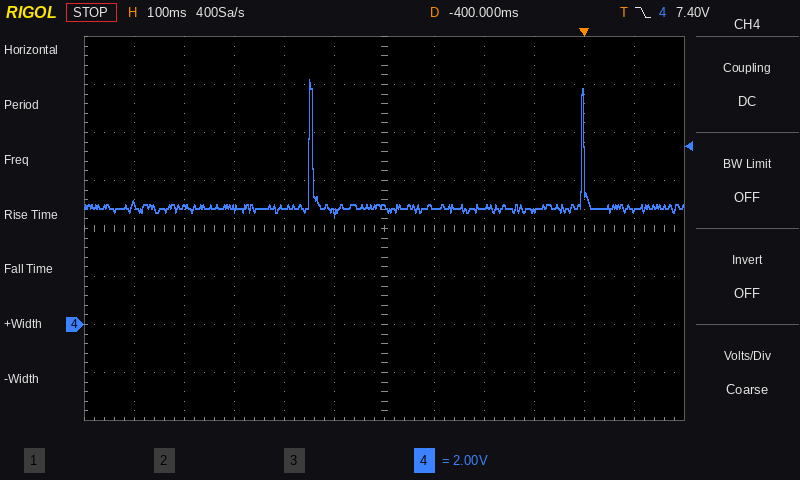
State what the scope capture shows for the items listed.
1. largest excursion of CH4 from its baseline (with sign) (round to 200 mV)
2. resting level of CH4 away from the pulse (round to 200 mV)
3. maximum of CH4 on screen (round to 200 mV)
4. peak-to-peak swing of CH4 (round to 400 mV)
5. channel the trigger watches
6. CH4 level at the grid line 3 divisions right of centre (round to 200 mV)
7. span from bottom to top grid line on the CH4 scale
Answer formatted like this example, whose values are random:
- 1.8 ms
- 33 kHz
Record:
- +5.4 V
- 4.8 V
- 10.2 V
- 5.6 V
- CH4
- 4.8 V
- 16 V
